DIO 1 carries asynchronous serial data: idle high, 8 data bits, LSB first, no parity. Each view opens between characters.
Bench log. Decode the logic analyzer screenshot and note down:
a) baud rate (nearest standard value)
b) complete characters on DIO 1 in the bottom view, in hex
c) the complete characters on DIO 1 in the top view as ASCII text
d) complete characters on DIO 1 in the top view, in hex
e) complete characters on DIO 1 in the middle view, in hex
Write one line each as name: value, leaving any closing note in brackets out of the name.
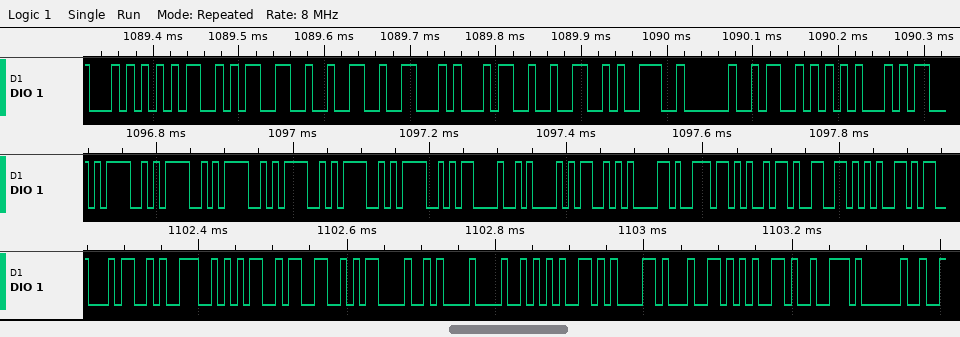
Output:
baud rate: 115200 baud
complete characters on DIO 1 in the bottom view, in hex: 34, 39, 35, 33, 0D, 0A, 48, 65, 61, 64, 65, 72, 20
the complete characters on DIO 1 in the top view as ASCII text: "TM32F429 SE"
complete characters on DIO 1 in the top view, in hex: 54, 4D, 33, 32, 46, 34, 32, 39, 20, 53, 45
complete characters on DIO 1 in the middle view, in hex: 3D, 3D, 3D, 3D, 3D, 3D, 0D, 0A, 4D, 61, 6E, 69, 66, 65
